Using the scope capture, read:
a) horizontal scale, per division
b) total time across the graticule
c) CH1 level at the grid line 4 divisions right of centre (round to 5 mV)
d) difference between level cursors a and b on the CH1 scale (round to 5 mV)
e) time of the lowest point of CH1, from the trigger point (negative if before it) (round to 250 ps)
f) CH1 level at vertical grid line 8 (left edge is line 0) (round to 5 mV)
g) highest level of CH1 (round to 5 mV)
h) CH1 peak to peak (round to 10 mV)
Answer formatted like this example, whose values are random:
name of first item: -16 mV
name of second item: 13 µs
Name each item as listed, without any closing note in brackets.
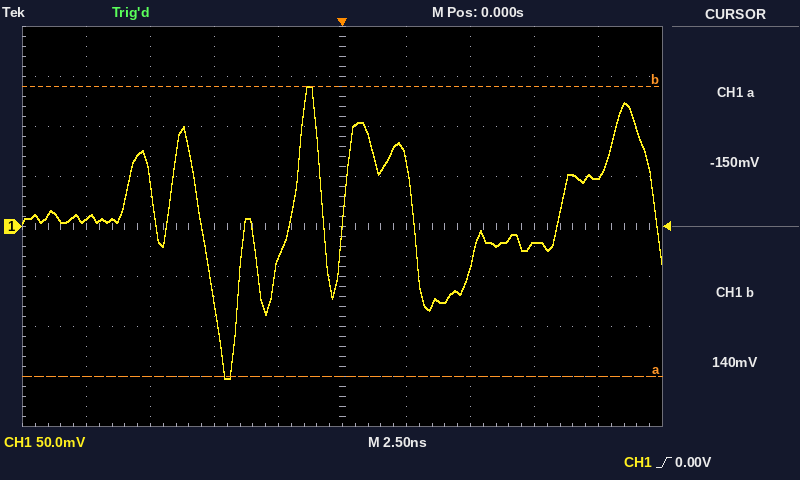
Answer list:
horizontal scale, per division: 2.5 ns
total time across the graticule: 25 ns
CH1 level at the grid line 4 divisions right of centre: 50 mV
difference between level cursors a and b on the CH1 scale: 290 mV
time of the lowest point of CH1, from the trigger point (negative if before it): -4.50 ns
CH1 level at vertical grid line 8 (left edge is line 0): -15 mV
highest level of CH1: 140 mV
CH1 peak to peak: 290 mV
